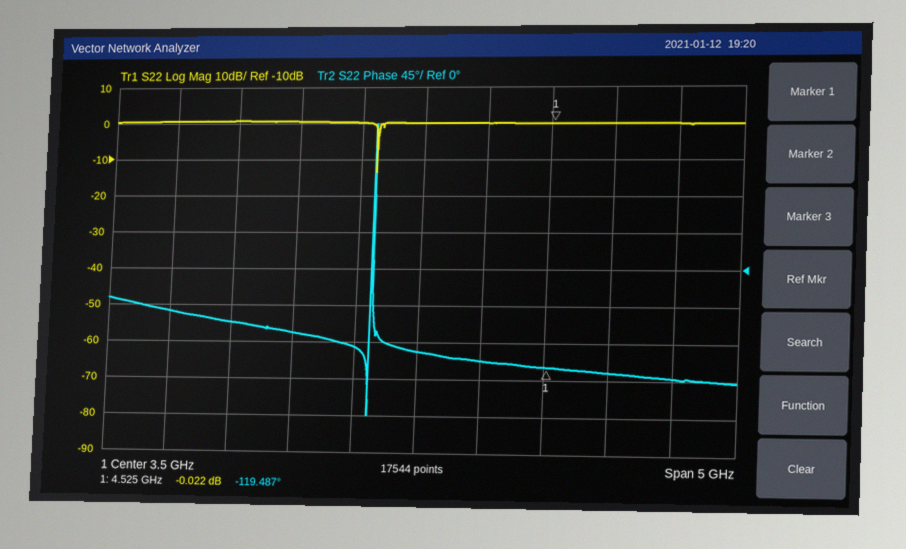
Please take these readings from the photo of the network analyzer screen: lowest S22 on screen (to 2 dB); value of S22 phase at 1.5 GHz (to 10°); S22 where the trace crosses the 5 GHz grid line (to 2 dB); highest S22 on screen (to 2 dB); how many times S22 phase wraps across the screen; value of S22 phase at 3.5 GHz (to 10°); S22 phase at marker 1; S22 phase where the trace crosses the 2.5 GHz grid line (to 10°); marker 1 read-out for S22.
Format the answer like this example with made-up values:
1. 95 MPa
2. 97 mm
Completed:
1. -14 dB
2. -50°
3. 0 dB
4. 0 dB
5. 1
6. -100°
7. -119.487°
8. -80°
9. -0.022 dB
